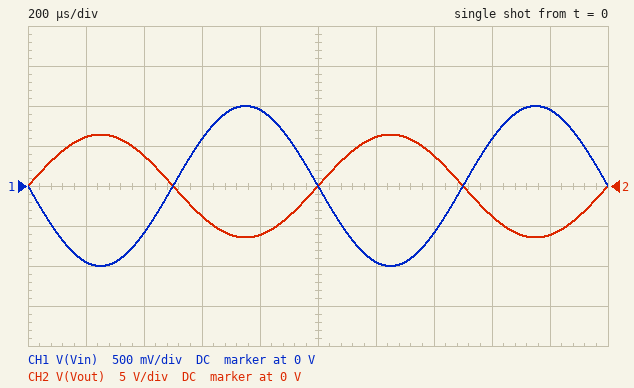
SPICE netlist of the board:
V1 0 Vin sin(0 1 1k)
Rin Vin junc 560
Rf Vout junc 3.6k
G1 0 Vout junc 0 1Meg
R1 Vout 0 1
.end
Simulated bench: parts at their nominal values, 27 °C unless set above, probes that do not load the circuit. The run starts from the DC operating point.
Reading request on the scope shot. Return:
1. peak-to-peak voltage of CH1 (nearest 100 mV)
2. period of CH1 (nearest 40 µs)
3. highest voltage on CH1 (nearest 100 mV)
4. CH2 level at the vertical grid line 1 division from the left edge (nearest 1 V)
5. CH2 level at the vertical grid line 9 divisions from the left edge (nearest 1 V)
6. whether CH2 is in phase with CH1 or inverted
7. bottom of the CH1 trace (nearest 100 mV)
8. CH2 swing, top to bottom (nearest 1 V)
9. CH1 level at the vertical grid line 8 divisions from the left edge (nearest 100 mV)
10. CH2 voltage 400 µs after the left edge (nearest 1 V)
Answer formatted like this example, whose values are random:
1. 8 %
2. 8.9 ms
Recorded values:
1. 2.0 V
2. 1.00 ms
3. 1.0 V
4. 6 V
5. -6 V
6. inverted
7. -1.0 V
8. 13 V
9. 600 mV
10. 4 V
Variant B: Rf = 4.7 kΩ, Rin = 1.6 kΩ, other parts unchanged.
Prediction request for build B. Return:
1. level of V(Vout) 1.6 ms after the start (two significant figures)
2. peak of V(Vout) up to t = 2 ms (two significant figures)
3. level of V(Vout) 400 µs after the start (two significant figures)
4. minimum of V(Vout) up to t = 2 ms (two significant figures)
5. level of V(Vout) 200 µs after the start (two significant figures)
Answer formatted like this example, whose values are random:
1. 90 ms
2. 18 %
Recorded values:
1. -1.7 V
2. 2.9 V
3. 1.7 V
4. -2.9 V
5. 2.8 V
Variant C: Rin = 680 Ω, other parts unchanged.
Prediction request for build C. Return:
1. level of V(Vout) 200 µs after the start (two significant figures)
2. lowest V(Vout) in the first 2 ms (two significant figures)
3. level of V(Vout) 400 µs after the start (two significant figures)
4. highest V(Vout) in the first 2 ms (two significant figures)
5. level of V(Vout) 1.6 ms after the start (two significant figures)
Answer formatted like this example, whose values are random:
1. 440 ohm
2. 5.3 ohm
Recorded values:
1. 5.0 V
2. -5.3 V
3. 3.1 V
4. 5.3 V
5. -3.1 V
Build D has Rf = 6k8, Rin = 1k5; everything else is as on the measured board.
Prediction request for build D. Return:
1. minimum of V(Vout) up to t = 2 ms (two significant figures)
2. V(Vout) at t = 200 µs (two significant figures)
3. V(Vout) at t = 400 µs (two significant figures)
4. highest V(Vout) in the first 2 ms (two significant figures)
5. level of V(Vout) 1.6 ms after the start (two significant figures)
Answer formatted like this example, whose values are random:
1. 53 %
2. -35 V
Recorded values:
1. -4.5 V
2. 4.3 V
3. 2.7 V
4. 4.5 V
5. -2.7 V
